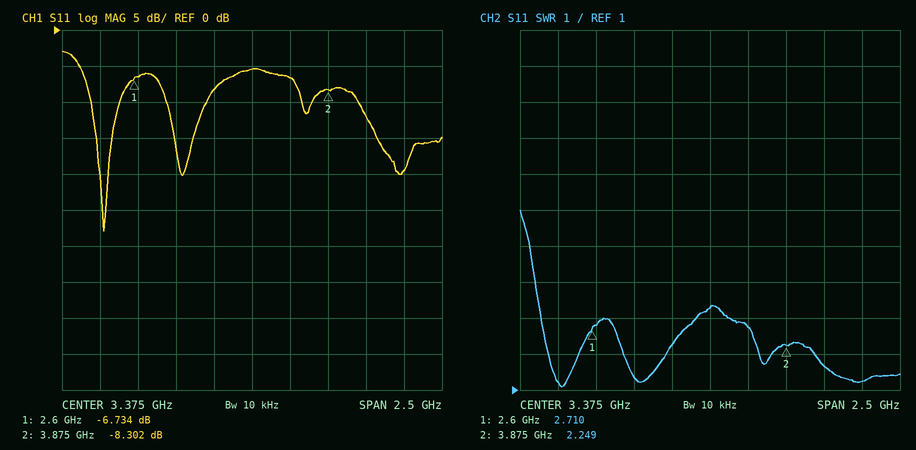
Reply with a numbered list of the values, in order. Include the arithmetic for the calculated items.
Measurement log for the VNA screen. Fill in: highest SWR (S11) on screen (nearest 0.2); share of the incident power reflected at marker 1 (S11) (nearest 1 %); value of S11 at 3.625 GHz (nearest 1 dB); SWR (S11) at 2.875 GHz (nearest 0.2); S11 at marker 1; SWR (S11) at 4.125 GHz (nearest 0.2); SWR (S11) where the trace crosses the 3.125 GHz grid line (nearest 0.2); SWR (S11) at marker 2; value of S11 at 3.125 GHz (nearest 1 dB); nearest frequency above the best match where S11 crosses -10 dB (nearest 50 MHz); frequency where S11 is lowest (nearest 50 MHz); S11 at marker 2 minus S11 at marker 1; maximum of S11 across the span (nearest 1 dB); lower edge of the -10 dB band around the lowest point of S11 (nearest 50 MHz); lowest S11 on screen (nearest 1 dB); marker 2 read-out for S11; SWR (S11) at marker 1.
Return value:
1. 6.0
2. 10^(-6.734/10) ≈ 21 %
3. -7 dB
4. 1.4
5. -6.734 dB
6. 1.6
7. 2.2
8. 2.249
9. -8 dB
10. 2.50 GHz
11. 2.40 GHz
12. -8.302 − (-6.734) = -1.568 dB
13. -3 dB
14. 2.30 GHz
15. -28 dB
16. -8.302 dB
17. 2.710
